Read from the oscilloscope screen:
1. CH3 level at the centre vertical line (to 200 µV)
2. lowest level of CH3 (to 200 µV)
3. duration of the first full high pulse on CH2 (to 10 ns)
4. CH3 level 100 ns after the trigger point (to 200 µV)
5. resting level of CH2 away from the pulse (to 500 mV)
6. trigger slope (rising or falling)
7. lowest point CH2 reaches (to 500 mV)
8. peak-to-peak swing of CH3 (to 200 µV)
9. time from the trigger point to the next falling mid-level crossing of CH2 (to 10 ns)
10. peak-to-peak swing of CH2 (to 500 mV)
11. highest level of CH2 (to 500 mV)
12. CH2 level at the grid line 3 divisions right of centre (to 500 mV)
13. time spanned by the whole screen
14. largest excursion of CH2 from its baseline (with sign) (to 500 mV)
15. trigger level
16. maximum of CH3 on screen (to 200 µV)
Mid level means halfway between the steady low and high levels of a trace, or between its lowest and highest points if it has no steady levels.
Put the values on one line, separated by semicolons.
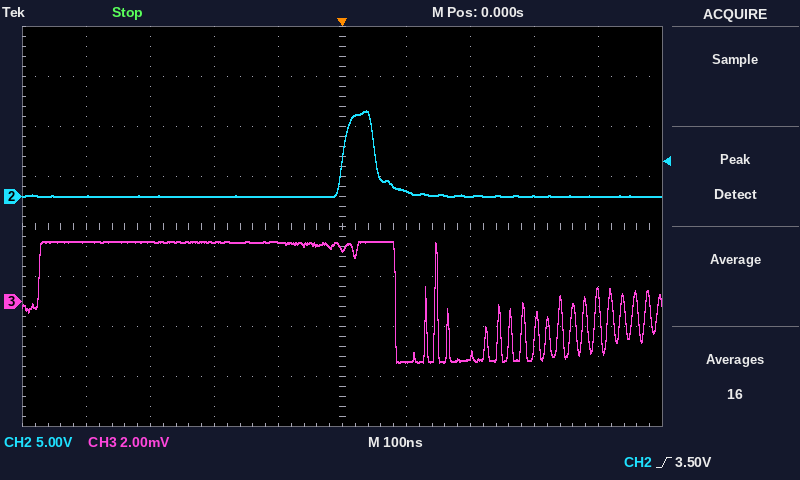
2.2 mV; -2.4 mV; 50 ns; -2.4 mV; 0.0 V; rising; 0.0 V; 4.8 mV; 50 ns; 8.5 V; 8.5 V; 0.0 V; 1 µs; +8.5 V; 3.50 V; 2.4 mV
